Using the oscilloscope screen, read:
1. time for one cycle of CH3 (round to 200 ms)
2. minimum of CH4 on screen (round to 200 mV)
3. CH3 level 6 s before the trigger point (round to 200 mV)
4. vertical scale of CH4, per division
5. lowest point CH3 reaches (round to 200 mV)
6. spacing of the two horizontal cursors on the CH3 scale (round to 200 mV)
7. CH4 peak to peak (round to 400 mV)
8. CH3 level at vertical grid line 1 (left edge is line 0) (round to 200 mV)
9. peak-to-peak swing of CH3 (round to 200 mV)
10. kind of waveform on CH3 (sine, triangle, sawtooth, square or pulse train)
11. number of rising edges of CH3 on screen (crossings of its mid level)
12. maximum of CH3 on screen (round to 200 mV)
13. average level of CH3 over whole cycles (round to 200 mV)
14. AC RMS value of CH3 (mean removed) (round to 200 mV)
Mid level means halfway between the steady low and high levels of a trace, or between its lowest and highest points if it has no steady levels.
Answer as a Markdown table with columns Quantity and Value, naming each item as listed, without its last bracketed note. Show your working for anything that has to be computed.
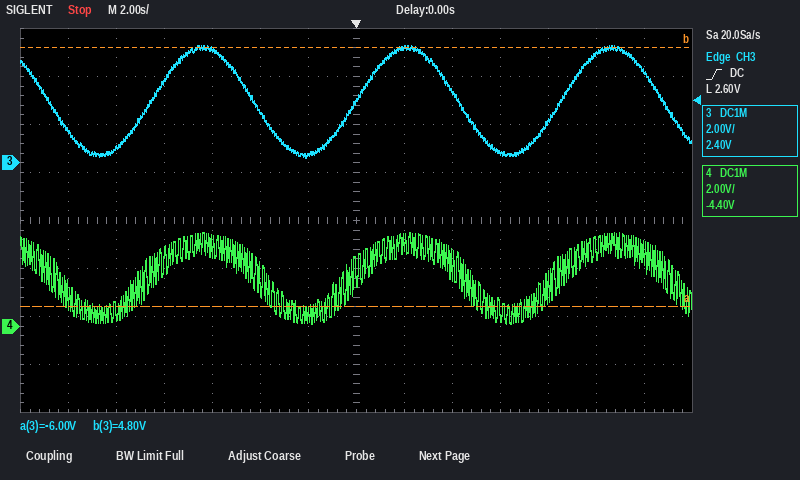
| Quantity | Value |
|---|---|
| time for one cycle of CH3 | 8.6 s |
| minimum of CH4 on screen | 200 mV |
| CH3 level 6 s before the trigger point | 4.8 V |
| vertical scale of CH4, per division | 2 V |
| lowest point CH3 reaches | 200 mV |
| spacing of the two horizontal cursors on the CH3 scale | 10.8 V |
| CH4 peak to peak | 3.6 V |
| CH3 level at vertical grid line 1 (left edge is line 0) | 1.4 V |
| peak-to-peak swing of CH3 | 4.8 V − (200 mV) = 4.6 V |
| kind of waveform on CH3 | sine |
| number of rising edges of CH3 on screen | 3 |
| maximum of CH3 on screen | 4.8 V |
| average level of CH3 over whole cycles | (4.8 V + (200 mV)) / 2 ≈ 2.50 V, so 2.6 V to the nearest 200 mV |
| AC RMS value of CH3 (mean removed) | 4.6 V / (2√2) ≈ 1.6 V |
